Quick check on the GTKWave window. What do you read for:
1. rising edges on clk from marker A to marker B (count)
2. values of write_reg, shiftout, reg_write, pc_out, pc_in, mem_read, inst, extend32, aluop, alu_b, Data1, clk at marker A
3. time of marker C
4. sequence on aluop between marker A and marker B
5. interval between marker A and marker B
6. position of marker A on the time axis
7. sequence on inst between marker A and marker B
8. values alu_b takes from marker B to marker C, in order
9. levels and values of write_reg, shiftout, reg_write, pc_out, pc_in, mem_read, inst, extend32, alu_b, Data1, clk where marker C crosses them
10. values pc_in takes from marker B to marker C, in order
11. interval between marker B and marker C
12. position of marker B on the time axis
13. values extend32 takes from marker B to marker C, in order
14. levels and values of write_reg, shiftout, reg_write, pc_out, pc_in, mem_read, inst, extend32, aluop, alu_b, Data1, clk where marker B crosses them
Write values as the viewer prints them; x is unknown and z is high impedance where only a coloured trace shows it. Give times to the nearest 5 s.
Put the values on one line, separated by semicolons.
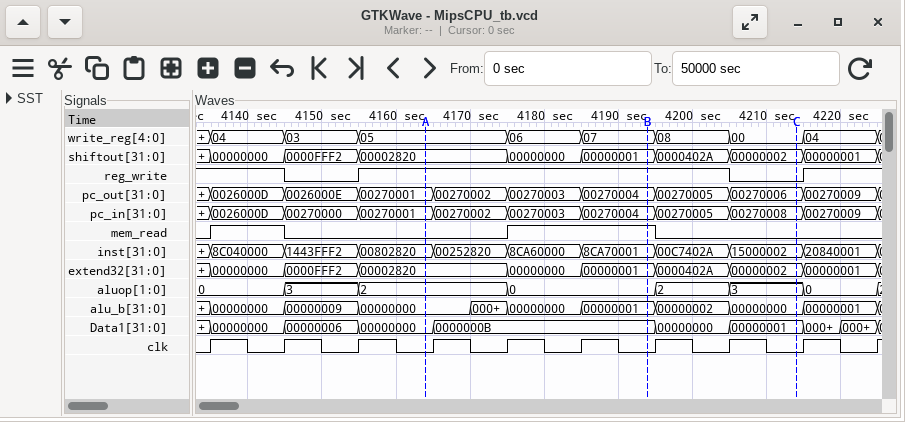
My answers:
3; write_reg=05, shiftout=00002820, reg_write=1, pc_out=00270001, pc_in=00270001, mem_read=0, inst=00802820, extend32=00002820, aluop=2, alu_b=00000000, Data1=00000000, clk=0; 4215 s; 2, 0; 30 s; 4165 s; 00802820, 00252820, 8CA60000, 8CA70001; 00000001, 00000002, 00000000; write_reg=00, shiftout=00000002, reg_write=0, pc_out=00270006, pc_in=00270008, mem_read=0, inst=15000002, extend32=00000002, alu_b=00000000, Data1=00000001, clk=0; 00270004, 00270005, 00270008; 20 s; 4195 s; 00000001, 0000402A, 00000002; write_reg=07, shiftout=00000001, reg_write=1, pc_out=00270004, pc_in=00270004, mem_read=1, inst=8CA70001, extend32=00000001, aluop=0, alu_b=00000001, Data1=0000000B, clk=0
